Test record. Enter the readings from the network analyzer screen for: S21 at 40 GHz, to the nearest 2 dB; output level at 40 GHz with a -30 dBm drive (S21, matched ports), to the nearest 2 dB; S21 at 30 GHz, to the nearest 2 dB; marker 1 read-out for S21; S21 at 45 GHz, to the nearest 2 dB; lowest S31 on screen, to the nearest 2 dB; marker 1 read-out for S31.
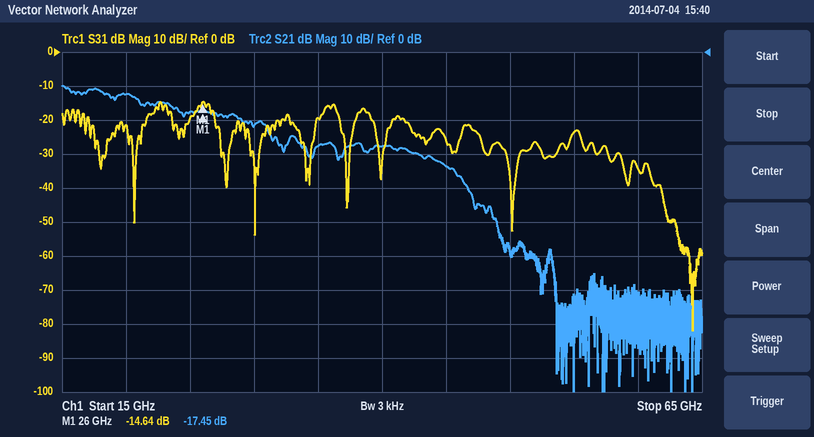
-28 dB
-58 dBm
-22 dB
-17.45 dB
-34 dB
-82 dB
-14.64 dB
